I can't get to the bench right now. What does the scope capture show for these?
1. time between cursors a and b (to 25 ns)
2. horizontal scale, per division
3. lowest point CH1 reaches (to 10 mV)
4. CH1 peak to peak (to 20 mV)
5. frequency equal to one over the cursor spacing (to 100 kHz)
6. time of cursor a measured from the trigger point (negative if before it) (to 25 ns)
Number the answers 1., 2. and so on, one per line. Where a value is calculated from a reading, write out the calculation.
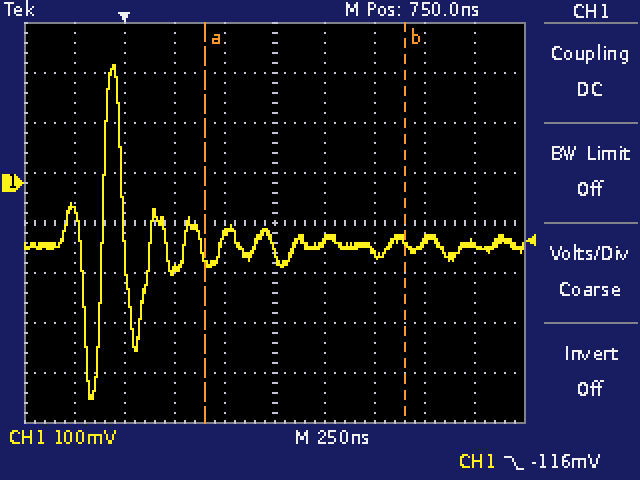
1. 1.000 µs
2. 250 ns
3. -430 mV
4. 660 mV
5. 1 / 1.000 µs ≈ 1.0 MHz
6. +400 ns
